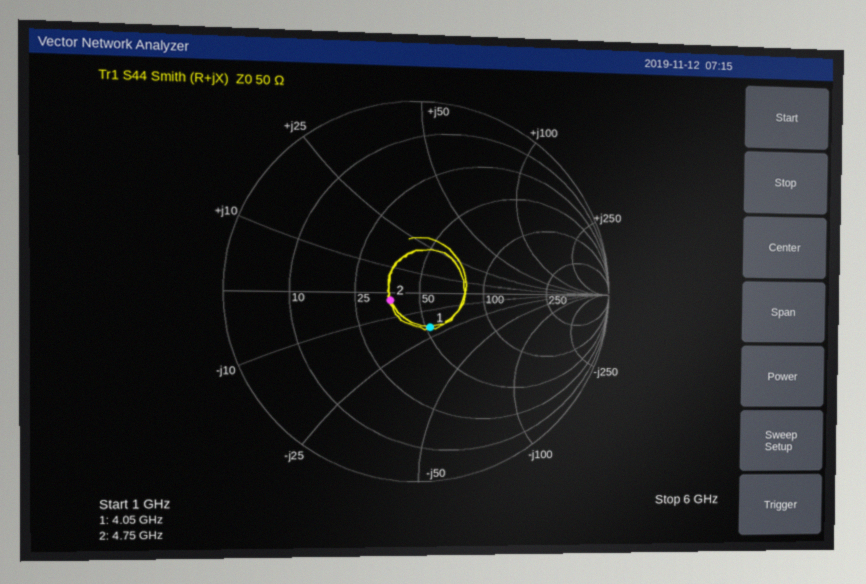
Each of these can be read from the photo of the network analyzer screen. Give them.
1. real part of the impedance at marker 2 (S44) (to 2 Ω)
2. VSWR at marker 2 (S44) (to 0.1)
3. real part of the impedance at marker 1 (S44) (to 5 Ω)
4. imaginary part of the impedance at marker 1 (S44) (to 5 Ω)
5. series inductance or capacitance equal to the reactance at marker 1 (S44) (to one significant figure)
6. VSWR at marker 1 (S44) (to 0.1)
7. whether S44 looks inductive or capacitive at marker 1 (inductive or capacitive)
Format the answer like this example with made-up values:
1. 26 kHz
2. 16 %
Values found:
1. 36 Ω
2. 1.4
3. 50 Ω
4. -20 Ω
5. 2 pF
6. 1.5
7. capacitive
